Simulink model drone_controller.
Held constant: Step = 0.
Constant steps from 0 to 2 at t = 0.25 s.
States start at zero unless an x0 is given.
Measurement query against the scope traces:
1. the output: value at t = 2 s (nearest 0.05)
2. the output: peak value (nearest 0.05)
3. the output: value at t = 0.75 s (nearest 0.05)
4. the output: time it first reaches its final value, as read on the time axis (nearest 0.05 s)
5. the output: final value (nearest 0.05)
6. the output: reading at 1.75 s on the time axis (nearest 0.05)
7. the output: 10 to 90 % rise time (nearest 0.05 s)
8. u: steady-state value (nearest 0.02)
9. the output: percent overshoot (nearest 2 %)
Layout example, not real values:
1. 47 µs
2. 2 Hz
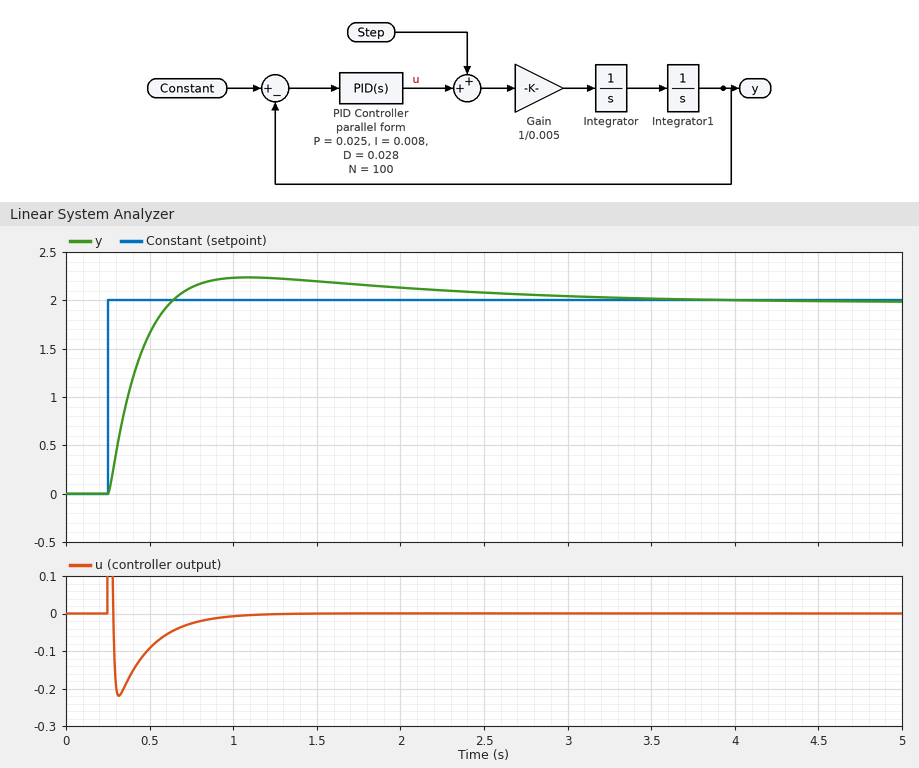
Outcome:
1. 2.15
2. 2.25
3. 2.15
4. 0.65 s
5. 2.00
6. 2.15
7. 0.25 s
8. 0.00
9. 12 %
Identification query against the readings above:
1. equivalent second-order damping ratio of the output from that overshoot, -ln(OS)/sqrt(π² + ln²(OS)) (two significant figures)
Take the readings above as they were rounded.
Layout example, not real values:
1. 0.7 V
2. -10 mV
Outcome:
1. 0.56
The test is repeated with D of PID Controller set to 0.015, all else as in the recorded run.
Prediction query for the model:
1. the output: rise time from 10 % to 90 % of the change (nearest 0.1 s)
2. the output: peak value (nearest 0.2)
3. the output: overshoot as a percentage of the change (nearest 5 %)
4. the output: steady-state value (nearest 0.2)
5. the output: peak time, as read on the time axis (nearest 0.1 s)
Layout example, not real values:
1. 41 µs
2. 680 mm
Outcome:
1. 0.4 s
2. 2.6
3. 25 %
4. 2.0
5. 1.3 s
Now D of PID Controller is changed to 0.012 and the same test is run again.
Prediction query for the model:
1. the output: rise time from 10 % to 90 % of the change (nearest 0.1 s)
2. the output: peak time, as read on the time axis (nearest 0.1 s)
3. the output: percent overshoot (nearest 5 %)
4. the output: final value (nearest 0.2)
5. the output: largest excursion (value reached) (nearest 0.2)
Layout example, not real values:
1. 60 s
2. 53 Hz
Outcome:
1. 0.4 s
2. 1.3 s
3. 35 %
4. 2.0
5. 2.6
